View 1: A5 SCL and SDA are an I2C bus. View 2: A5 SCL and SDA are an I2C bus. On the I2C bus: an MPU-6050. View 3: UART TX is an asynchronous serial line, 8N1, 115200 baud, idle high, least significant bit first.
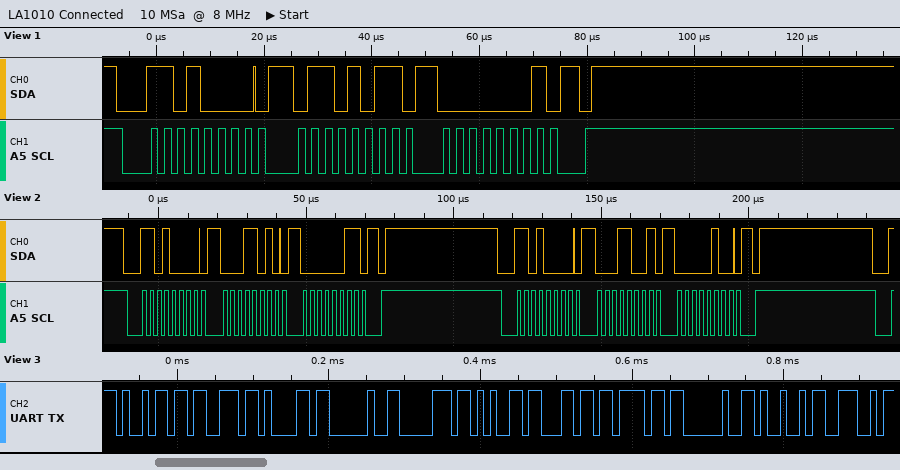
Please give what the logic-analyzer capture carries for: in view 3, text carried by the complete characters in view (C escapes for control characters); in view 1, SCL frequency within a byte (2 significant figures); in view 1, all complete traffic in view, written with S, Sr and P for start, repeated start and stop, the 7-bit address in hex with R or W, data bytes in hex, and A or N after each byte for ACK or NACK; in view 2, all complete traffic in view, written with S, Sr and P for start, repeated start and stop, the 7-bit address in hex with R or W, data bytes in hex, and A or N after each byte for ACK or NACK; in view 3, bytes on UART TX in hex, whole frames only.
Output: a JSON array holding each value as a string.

["\"isa pelo IN\"", "400 kHz", "S 68W A 6B A 01 A P", "S 68W A 1A A 03 A P S 68W A 19 A 04 A P", "69 73 61 20 70 65 6C 6F 20 49 4E"]
